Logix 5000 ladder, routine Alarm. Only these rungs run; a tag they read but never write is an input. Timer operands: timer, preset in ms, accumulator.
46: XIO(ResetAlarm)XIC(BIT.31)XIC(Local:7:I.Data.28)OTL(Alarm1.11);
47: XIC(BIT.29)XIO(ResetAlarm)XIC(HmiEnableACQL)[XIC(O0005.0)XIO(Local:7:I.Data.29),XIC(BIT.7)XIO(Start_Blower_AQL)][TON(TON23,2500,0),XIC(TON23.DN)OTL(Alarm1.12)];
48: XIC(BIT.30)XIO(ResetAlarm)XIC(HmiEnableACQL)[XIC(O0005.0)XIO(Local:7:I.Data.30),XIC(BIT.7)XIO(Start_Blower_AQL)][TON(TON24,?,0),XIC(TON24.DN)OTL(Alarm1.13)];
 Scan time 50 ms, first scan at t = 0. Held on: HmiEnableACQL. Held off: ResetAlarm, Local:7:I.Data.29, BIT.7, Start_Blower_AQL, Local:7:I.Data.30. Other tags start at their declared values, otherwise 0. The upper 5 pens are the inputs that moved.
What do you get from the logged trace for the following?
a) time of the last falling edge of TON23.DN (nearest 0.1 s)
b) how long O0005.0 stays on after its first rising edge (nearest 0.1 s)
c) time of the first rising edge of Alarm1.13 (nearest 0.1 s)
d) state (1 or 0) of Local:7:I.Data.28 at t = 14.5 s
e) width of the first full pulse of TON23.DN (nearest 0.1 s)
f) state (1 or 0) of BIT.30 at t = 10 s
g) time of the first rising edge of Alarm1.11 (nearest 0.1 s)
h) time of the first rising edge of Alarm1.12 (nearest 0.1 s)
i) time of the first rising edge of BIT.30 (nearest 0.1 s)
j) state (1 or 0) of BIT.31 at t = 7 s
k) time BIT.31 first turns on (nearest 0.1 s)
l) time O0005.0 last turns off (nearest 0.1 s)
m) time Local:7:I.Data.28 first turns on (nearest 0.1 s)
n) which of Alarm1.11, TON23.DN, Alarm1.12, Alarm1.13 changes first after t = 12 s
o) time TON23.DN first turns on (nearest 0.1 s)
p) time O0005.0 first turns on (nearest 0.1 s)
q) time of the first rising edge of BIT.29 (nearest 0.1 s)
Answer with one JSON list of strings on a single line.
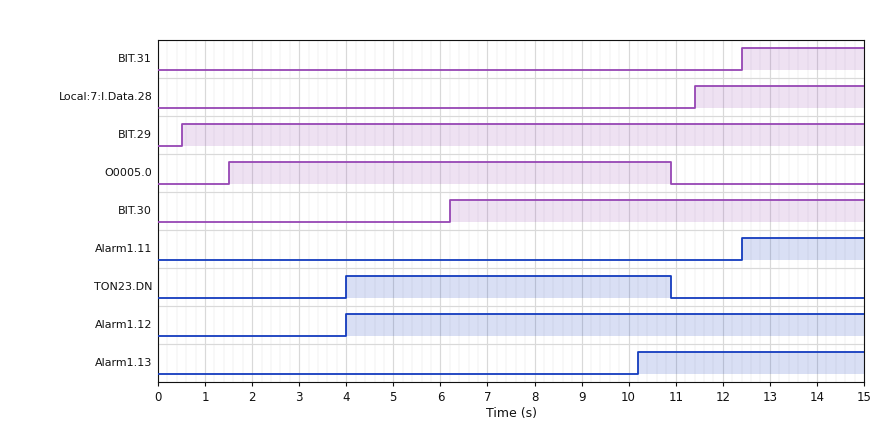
["10.9 s", "9.4 s", "10.2 s", "1", "6.9 s", "1", "12.4 s", "4.0 s", "6.2 s", "0", "12.4 s", "10.9 s", "11.4 s", "Alarm1.11", "4.0 s", "1.5 s", "0.5 s"]
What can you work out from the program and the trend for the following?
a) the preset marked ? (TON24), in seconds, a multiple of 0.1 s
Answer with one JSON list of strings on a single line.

["4.0 s"]
